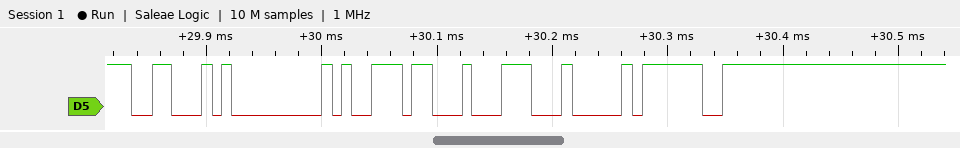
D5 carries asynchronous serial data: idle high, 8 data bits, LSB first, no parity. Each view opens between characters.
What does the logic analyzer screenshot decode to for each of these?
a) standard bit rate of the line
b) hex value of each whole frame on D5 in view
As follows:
115200 baud
46, 00, B9, C4, 04, 3F
